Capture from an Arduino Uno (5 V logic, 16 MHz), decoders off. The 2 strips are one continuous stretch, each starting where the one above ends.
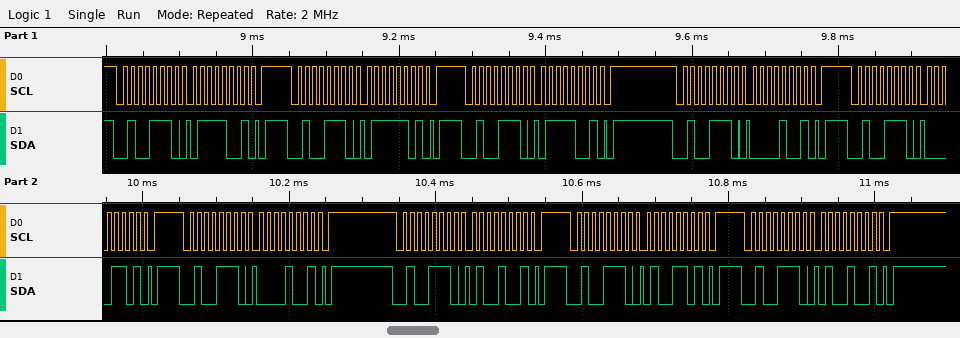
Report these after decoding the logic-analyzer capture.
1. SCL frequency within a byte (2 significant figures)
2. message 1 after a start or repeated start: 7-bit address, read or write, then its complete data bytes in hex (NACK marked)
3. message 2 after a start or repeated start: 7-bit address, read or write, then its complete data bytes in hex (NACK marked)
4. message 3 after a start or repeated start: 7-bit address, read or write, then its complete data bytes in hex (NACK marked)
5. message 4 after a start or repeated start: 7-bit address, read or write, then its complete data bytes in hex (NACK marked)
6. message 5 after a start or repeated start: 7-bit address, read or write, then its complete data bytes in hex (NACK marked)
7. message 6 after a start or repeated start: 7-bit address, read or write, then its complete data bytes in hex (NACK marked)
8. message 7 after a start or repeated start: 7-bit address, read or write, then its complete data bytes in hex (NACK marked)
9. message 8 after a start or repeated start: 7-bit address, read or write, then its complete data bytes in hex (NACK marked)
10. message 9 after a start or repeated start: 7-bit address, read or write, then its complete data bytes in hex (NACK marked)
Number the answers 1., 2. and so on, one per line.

1. 100 kHz
2. 0x27 write: 79
3. 0x27 write: 7D
4. 0x27 write: 79
5. 0x27 write: 09
6. 0x27 write: 0D
7. 0x27 write: 09
8. 0x27 write: 49
9. 0x27 write: 4D
10. 0x27 write: 49
